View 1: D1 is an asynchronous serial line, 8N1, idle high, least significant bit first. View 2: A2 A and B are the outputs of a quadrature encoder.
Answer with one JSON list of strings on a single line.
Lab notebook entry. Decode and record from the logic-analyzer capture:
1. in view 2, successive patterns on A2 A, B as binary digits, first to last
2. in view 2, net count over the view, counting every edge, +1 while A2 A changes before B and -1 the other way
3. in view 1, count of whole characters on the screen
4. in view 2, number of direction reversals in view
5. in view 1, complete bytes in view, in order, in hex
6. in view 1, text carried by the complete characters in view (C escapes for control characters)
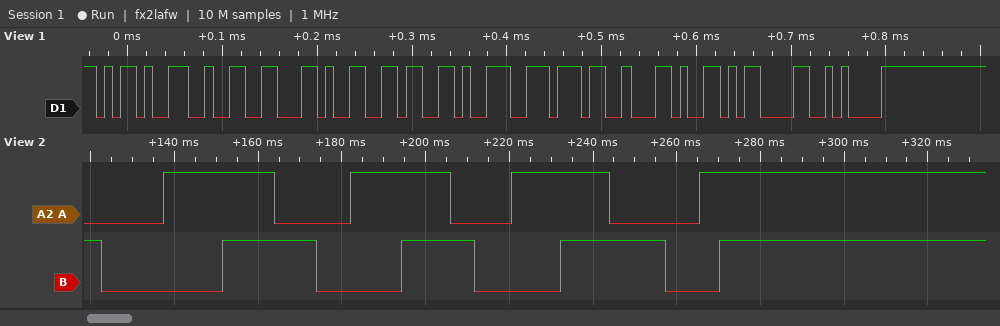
["01 00 10 11 01 00 10 11 01 00 10 11 01 00 10 11", "+15", "9", "0", "2D 32 2C 36 39 37 2C 0D 0A", "\"-2,697,\\r\\n\""]
